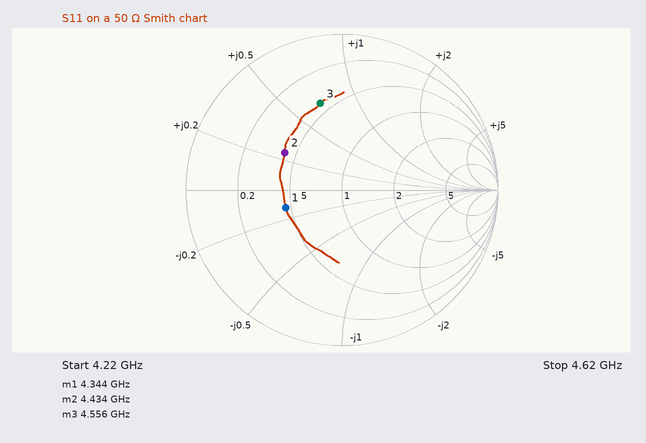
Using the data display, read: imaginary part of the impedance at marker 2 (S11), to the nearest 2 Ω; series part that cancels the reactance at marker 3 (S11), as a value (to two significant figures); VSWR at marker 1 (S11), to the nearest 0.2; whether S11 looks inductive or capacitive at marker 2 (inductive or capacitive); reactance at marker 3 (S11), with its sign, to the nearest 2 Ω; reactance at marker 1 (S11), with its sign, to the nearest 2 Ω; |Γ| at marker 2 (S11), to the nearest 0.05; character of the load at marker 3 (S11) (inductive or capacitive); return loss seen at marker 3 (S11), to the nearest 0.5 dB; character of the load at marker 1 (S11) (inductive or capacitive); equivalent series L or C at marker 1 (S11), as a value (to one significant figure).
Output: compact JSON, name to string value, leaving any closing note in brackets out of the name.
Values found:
{"imaginary part of the impedance at marker 2 (S11), to the nearest 2 Ω": "+12 Ω", "series part that cancels the reactance at marker 3 (S11), as a value": "1.0 pF", "VSWR at marker 1 (S11), to the nearest 0.2": "2.2", "whether S11 looks inductive or capacitive at marker 2": "inductive", "reactance at marker 3 (S11), with its sign, to the nearest 2 Ω": "+34 Ω", "reactance at marker 1 (S11), with its sign, to the nearest 2 Ω": "-6 Ω", "|Γ| at marker 2 (S11), to the nearest 0.05": "0.45", "character of the load at marker 3 (S11)": "inductive", "return loss seen at marker 3 (S11), to the nearest 0.5 dB": "5.0 dB", "character of the load at marker 1 (S11)": "capacitive", "equivalent series L or C at marker 1 (S11), as a value": "6 pF"}
